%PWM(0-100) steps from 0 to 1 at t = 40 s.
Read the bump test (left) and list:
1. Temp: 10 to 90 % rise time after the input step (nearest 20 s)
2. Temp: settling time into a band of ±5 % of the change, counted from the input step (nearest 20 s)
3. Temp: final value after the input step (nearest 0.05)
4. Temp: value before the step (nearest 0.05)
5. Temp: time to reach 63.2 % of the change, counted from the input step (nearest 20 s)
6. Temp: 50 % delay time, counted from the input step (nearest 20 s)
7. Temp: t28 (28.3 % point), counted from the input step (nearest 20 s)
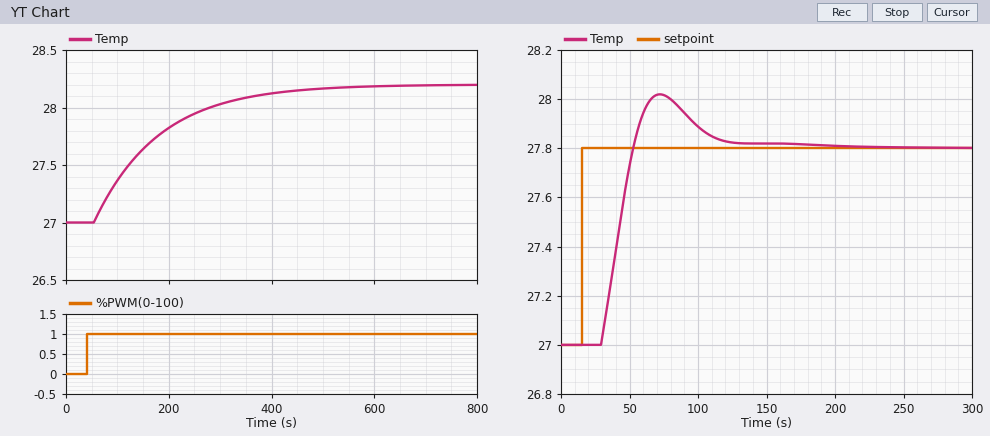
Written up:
280 s
400 s
28.20
27.00
140 s
100 s
60 s
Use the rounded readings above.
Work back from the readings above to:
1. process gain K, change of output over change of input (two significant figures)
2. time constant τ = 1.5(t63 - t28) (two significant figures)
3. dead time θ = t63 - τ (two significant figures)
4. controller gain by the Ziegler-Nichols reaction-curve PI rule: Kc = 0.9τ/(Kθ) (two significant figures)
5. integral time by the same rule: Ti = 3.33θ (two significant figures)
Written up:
1.2
120 s
20 s
4.5
67 s
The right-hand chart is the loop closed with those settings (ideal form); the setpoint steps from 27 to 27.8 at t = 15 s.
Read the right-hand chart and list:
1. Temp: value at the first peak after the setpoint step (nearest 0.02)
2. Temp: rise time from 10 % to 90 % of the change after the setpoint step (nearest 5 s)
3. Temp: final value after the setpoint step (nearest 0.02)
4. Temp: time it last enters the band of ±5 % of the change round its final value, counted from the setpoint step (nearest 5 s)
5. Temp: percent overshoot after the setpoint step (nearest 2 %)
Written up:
28.02
20 s
27.80
100 s
28 %
